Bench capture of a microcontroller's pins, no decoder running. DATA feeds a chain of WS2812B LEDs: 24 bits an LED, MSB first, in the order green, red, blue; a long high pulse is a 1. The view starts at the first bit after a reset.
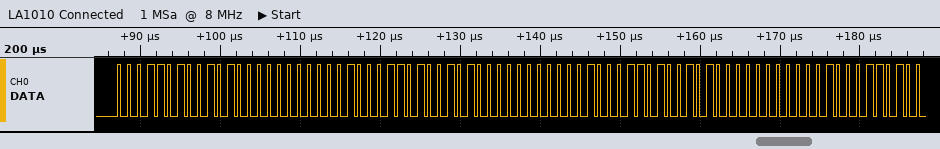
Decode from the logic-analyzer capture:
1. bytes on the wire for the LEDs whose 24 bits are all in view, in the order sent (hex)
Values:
1A 50 01 1A 50 01 1A 50 01
